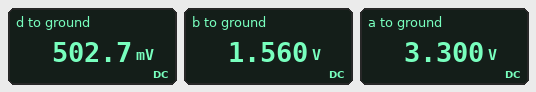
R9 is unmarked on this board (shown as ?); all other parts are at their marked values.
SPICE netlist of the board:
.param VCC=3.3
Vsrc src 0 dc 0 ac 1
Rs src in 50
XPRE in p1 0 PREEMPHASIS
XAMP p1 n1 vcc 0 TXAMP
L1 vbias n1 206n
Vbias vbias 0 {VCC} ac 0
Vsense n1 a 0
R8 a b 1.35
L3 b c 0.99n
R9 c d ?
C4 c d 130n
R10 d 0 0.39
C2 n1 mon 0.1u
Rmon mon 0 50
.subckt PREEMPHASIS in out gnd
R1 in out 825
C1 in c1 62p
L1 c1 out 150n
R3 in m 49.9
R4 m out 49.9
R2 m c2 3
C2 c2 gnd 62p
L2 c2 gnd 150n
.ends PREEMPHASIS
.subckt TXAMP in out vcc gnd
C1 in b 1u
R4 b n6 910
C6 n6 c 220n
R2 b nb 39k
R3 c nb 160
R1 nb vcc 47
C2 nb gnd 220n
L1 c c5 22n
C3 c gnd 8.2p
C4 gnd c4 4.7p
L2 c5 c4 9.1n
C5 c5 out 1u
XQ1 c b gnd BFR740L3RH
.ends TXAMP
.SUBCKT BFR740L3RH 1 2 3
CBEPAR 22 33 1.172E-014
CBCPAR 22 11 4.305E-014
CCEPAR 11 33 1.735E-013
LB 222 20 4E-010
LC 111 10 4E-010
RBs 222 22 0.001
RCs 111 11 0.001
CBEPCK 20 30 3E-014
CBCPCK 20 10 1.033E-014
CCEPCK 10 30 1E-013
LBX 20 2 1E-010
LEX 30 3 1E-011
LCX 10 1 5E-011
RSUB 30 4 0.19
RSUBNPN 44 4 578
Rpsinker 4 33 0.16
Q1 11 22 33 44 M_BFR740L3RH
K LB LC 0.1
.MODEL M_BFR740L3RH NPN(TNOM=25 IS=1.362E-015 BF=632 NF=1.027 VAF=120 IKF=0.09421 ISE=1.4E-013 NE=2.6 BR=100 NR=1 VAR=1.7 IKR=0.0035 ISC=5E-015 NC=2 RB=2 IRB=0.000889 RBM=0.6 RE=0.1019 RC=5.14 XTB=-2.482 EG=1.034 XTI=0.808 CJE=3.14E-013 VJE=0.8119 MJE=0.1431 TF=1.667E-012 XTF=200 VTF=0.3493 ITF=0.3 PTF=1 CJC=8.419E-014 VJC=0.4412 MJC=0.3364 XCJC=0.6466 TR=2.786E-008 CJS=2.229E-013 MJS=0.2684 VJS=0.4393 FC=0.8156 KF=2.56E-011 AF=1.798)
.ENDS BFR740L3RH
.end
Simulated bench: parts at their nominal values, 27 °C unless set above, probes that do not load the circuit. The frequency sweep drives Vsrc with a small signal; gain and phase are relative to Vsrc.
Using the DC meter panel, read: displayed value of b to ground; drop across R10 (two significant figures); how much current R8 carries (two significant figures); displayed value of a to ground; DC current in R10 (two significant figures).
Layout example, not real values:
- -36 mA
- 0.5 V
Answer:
- 1.560 V
- 500 mV
- 1.3 A
- 3.300 V
- 1.3 A
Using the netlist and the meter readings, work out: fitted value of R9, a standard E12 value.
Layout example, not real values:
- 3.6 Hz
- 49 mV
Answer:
- 0.82 Ω
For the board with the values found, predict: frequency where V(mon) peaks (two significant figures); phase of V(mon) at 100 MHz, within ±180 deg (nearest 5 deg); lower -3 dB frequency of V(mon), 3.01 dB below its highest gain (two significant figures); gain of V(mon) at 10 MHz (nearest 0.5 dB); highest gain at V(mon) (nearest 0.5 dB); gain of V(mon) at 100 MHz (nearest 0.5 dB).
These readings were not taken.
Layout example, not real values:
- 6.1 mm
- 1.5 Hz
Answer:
- 53 MHz
- -35 deg
- 34 MHz
- -69.5 dB
- -55.0 dB
- -59.0 dB
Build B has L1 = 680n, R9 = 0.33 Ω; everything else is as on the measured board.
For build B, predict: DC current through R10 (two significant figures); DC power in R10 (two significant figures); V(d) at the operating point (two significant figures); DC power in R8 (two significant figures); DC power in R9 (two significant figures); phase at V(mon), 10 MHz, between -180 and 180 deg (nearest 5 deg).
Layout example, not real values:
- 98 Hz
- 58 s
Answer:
- 1.6 A
- 990 mW
- 620 mV
- 3.4 W
- 840 mW
- 65 deg
